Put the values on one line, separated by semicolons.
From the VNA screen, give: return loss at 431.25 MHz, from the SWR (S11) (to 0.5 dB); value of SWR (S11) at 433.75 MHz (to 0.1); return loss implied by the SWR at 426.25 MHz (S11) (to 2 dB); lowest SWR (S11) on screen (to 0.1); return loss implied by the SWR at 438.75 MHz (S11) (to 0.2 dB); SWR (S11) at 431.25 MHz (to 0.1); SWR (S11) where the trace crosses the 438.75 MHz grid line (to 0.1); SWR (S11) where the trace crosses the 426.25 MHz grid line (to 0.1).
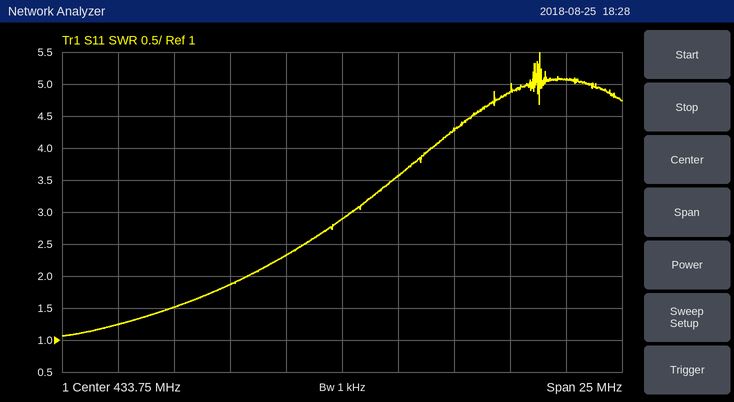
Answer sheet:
8.0 dB; 2.9; 14 dB; 1.1; 4.2 dB; 2.3; 4.3; 1.5
